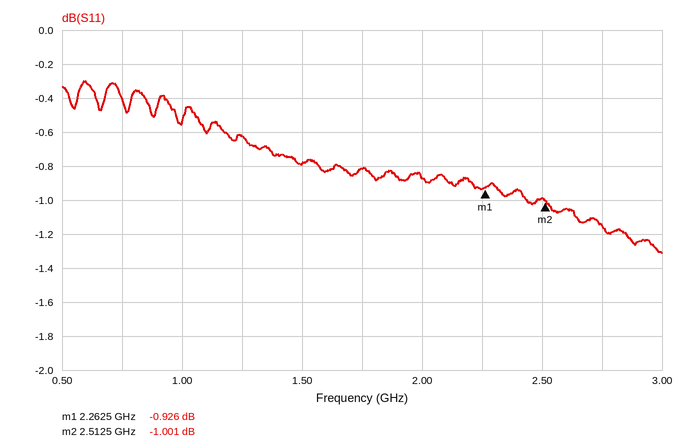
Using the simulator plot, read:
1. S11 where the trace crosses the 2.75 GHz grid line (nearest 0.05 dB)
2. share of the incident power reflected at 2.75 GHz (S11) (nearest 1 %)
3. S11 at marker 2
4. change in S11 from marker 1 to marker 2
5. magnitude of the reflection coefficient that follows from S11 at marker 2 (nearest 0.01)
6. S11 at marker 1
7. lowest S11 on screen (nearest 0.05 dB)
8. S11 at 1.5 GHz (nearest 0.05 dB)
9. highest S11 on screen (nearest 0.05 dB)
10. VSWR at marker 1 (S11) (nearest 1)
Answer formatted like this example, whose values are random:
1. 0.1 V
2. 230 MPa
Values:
1. -1.15 dB
2. 77 %
3. -1.001 dB
4. -0.075 dB
5. 0.89
6. -0.926 dB
7. -1.30 dB
8. -0.80 dB
9. -0.30 dB
10. 19
